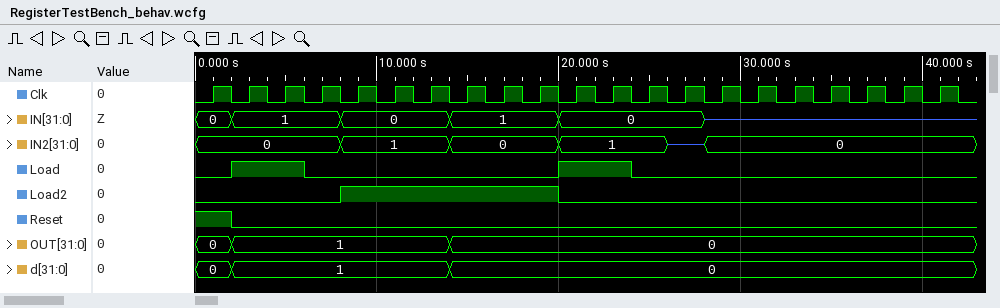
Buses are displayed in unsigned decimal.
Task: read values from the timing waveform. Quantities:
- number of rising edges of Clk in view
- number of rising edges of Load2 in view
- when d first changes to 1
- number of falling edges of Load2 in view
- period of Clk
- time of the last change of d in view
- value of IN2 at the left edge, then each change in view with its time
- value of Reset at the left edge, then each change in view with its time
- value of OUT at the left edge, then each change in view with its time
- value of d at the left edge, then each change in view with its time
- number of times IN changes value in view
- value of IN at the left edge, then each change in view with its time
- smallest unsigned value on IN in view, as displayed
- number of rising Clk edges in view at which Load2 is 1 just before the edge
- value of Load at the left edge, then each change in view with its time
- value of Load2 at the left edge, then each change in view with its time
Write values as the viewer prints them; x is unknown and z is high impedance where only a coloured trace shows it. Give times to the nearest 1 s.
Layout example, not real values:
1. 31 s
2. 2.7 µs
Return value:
1. 21
2. 1
3. 2 s
4. 1
5. 2 s
6. 14 s
7. 0, 1 at 8 s, 0 at 14 s, 1 at 20 s, z at 26 s, 0 at 28 s
8. 1, 0 at 2 s
9. 0, 1 at 2 s, 0 at 14 s
10. 0, 1 at 2 s, 0 at 14 s
11. 5
12. 0, 1 at 2 s, 0 at 8 s, 1 at 14 s, 0 at 20 s, z at 28 s
13. 0
14. 6
15. 0, 1 at 2 s, 0 at 6 s, 1 at 20 s, 0 at 24 s
16. 0, 1 at 8 s, 0 at 20 s
